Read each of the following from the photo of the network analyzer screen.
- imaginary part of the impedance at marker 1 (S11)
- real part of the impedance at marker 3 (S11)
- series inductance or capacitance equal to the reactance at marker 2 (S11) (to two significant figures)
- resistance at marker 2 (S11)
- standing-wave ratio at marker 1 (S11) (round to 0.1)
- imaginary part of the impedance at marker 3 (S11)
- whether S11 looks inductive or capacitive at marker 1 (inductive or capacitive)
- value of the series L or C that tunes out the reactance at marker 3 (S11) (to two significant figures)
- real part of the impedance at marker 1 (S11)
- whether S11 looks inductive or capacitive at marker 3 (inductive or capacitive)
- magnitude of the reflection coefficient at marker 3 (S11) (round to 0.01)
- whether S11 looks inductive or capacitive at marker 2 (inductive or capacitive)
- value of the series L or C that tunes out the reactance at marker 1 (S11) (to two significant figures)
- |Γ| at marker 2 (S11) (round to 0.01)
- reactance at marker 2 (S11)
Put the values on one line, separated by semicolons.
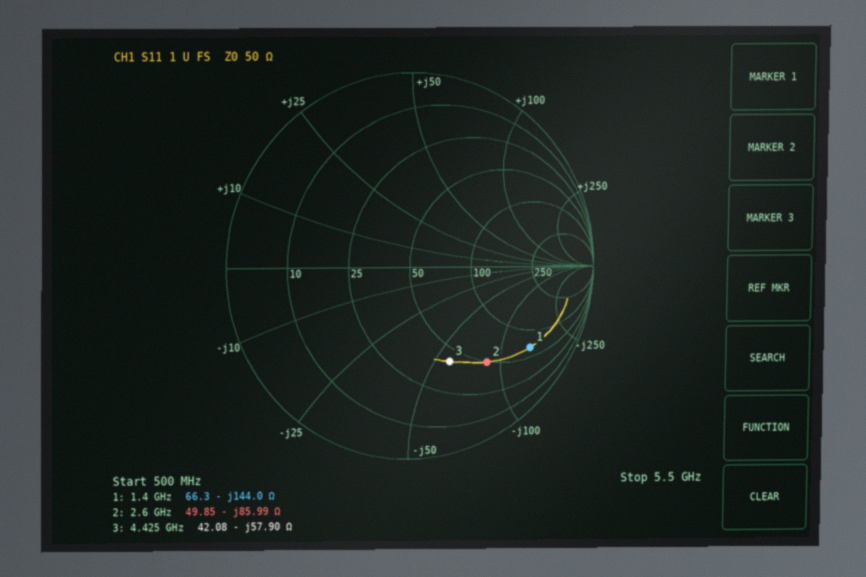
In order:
-144.0 Ω; 42.08 Ω; 710 fF; 49.85 Ω; 8.2; -57.90 Ω; capacitive; 2.1 nH; 66.3 Ω; capacitive; 0.54; capacitive; 16 nH; 0.65; -85.99 Ω
